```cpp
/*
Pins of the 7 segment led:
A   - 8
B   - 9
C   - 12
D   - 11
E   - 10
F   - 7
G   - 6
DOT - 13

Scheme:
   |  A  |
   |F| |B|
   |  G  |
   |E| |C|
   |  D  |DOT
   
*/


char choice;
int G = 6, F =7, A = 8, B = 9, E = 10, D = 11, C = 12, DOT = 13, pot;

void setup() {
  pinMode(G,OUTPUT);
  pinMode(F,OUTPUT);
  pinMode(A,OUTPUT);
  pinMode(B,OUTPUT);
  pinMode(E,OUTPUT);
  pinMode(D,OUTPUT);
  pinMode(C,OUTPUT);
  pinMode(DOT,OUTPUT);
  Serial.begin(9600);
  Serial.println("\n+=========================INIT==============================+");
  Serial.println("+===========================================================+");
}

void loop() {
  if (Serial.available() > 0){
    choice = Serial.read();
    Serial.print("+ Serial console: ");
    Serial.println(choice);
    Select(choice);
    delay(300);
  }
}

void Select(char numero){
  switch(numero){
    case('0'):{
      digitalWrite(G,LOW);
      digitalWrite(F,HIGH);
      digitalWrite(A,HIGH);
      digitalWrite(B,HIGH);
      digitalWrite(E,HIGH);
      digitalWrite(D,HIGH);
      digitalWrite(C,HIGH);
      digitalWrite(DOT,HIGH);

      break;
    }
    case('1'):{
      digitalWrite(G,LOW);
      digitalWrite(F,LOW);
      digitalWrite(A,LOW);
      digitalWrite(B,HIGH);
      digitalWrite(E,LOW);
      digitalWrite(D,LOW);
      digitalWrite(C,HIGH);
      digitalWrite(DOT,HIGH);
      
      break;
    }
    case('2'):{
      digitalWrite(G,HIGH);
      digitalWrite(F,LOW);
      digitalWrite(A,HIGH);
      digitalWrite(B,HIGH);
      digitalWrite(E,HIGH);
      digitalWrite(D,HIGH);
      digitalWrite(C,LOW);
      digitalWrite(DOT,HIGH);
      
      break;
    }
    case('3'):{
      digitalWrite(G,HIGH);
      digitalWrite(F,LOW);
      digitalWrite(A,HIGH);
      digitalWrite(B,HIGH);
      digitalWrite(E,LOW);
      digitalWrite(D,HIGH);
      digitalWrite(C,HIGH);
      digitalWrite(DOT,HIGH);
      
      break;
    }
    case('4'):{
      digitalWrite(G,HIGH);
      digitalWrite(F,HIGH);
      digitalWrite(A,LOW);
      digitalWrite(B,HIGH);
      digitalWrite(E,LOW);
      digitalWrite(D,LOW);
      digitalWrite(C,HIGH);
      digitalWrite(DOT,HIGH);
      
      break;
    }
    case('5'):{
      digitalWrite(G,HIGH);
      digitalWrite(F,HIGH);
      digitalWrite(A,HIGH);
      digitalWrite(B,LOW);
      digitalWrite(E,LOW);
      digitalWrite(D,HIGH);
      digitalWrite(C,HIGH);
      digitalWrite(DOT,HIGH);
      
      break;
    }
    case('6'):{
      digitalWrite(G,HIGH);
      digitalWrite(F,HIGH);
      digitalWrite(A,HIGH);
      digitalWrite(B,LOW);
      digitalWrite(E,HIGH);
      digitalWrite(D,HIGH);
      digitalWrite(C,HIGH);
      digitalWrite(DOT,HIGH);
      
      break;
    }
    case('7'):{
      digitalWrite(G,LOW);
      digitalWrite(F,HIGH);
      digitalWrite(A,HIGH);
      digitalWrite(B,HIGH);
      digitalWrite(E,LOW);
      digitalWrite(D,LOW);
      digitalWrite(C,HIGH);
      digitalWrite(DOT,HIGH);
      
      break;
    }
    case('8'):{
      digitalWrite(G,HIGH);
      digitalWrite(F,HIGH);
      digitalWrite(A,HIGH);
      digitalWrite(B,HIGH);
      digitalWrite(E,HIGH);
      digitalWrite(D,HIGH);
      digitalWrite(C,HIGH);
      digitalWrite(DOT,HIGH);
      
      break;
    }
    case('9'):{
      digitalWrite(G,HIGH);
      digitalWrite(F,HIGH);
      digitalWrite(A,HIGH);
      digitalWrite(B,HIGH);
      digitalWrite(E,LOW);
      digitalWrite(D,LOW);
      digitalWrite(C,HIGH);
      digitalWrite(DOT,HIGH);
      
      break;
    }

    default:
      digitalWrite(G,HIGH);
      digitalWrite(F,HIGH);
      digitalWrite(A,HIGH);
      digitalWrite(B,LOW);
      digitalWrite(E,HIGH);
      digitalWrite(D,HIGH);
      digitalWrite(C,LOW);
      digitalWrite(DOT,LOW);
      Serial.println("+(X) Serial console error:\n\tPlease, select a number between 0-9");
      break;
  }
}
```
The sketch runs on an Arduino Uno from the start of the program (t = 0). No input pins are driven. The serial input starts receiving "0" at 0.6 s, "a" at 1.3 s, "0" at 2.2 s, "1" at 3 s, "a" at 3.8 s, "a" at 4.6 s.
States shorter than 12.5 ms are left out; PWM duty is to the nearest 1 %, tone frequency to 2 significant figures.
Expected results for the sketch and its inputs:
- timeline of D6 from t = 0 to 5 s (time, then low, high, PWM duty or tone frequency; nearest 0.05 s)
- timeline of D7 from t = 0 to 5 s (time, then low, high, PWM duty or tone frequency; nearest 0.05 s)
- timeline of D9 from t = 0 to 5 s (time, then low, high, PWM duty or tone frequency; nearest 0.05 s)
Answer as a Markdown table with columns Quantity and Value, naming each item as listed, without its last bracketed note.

| Quantity | Value |
|---|---|
| timeline of D6 from t = 0 to 5 s | 0 s low; 1.3 s high; 2.2 s low; 3.8 s high |
| timeline of D7 from t = 0 to 5 s | 0 s low; 0.6 s high; 3 s low; 3.8 s high |
| timeline of D9 from t = 0 to 5 s | 0 s low; 0.6 s high; 1.3 s low; 2.2 s high; 3.8 s low |
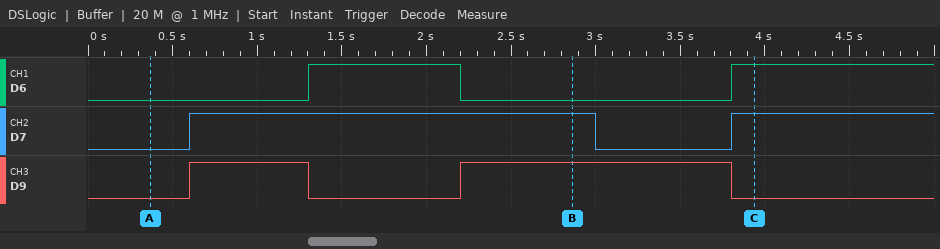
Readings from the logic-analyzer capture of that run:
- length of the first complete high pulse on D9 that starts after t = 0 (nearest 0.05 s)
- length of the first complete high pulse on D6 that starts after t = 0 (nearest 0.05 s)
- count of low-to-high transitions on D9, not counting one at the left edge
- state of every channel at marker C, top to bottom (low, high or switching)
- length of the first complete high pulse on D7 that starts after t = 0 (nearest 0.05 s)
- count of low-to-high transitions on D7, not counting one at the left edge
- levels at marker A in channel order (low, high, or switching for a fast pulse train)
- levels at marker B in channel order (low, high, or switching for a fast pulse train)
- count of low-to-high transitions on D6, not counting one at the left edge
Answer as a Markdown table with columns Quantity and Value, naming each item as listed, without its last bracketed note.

| Quantity | Value |
|---|---|
| length of the first complete high pulse on D9 that starts after t = 0 | 0.70 s |
| length of the first complete high pulse on D6 that starts after t = 0 | 0.90 s |
| count of low-to-high transitions on D9, not counting one at the left edge | 2 |
| state of every channel at marker C, top to bottom | D6 high, D7 high, D9 low |
| length of the first complete high pulse on D7 that starts after t = 0 | 2.40 s |
| count of low-to-high transitions on D7, not counting one at the left edge | 2 |
| levels at marker A in channel order | D6 low, D7 low, D9 low |
| levels at marker B in channel order | D6 low, D7 high, D9 high |
| count of low-to-high transitions on D6, not counting one at the left edge | 2 |
